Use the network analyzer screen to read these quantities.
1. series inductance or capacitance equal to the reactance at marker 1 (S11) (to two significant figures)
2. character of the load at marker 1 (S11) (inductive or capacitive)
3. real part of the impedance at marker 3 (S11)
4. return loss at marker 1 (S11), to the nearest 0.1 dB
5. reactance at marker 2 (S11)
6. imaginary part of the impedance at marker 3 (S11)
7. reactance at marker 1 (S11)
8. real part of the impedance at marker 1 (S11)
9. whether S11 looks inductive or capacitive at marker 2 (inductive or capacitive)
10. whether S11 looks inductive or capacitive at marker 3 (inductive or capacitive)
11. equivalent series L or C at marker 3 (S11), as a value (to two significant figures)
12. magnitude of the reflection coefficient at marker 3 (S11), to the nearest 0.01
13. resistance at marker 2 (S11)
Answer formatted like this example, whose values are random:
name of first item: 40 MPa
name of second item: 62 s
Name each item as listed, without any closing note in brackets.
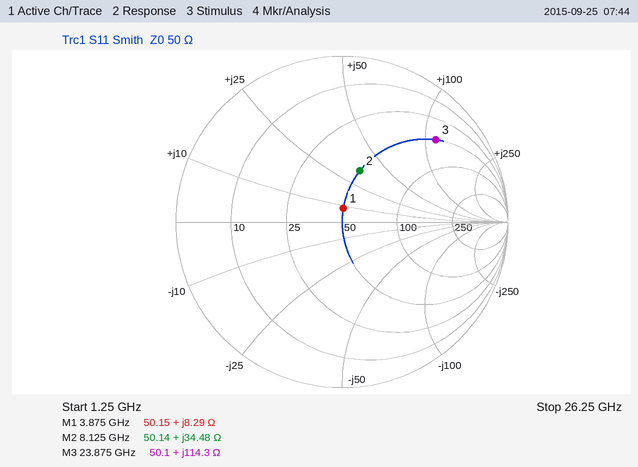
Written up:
series inductance or capacitance equal to the reactance at marker 1 (S11): 340 pH
character of the load at marker 1 (S11): inductive
real part of the impedance at marker 3: 50.1 Ω
return loss at marker 1 (S11), to the nearest 0.1 dB: 21.7 dB
reactance at marker 2: +34.48 Ω
imaginary part of the impedance at marker 3: +114.3 Ω
reactance at marker 1: +8.29 Ω
real part of the impedance at marker 1: 50.15 Ω
whether S11 looks inductive or capacitive at marker 2: inductive
whether S11 looks inductive or capacitive at marker 3: inductive
equivalent series L or C at marker 3 (S11), as a value: 760 pH
magnitude of the reflection coefficient at marker 3 (S11), to the nearest 0.01: 0.75
resistance at marker 2: 50.14 Ω
